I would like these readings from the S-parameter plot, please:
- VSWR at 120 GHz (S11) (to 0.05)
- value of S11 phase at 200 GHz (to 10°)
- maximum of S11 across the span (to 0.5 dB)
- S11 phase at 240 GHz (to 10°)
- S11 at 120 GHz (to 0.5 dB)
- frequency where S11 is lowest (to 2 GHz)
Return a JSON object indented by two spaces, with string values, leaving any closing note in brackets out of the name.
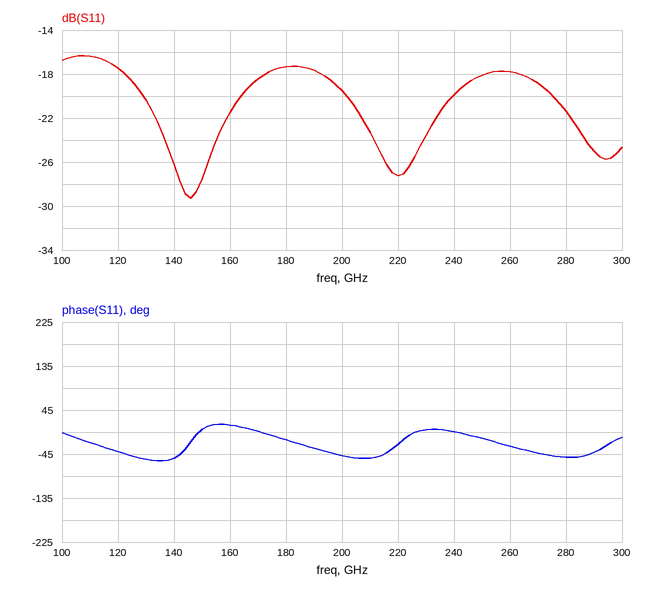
{
  "VSWR at 120 GHz (S11)": "1.30",
  "value of S11 phase at 200 GHz": "-50°",
  "maximum of S11 across the span": "-16.5 dB",
  "S11 phase at 240 GHz": "0°",
  "S11 at 120 GHz": "-17.5 dB",
  "frequency where S11 is lowest": "146 GHz"
}
